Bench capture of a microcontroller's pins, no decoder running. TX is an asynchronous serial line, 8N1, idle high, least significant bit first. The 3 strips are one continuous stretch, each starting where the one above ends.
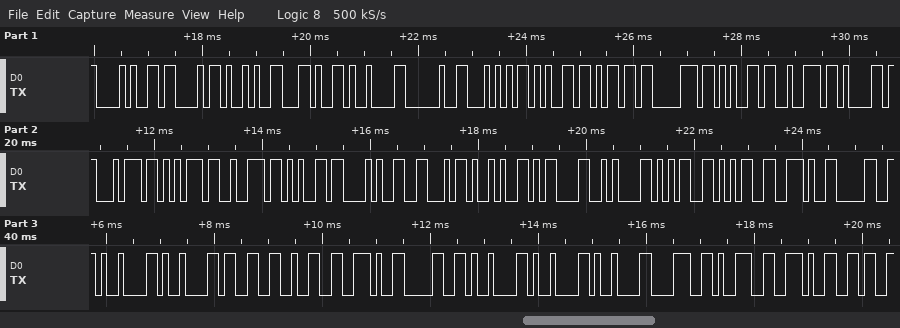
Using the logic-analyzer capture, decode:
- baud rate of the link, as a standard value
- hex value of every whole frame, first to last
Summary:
9600 baud
28 43 29 2C 09 20 54 65 6D 70 65 72 61 74 75 72 65 28 46 29 0D 0A 35 35 2E 30 09 09 33 32 2E 30 09 09 09 38 39 2E 36
